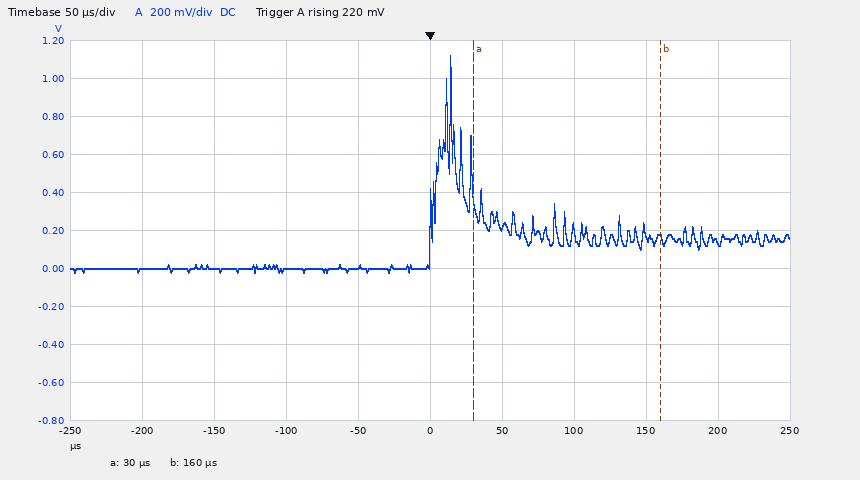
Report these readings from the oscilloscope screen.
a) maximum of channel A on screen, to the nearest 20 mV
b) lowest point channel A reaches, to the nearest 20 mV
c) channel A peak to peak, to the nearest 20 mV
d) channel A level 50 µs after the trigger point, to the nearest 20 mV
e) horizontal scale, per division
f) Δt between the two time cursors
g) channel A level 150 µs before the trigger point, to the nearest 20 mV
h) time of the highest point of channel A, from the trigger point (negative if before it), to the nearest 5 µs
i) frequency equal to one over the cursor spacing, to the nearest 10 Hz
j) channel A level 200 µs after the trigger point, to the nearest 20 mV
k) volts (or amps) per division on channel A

1.12 V
-20 mV
1.14 V
220 mV
50 µs
130 µs
0 mV
+15 µs
7.69 kHz
140 mV
200 mV
